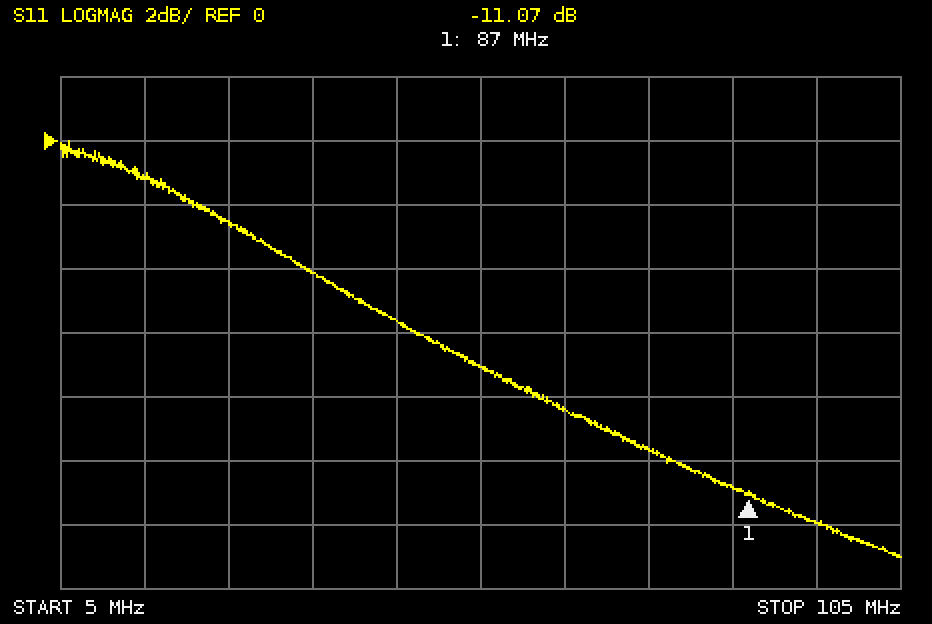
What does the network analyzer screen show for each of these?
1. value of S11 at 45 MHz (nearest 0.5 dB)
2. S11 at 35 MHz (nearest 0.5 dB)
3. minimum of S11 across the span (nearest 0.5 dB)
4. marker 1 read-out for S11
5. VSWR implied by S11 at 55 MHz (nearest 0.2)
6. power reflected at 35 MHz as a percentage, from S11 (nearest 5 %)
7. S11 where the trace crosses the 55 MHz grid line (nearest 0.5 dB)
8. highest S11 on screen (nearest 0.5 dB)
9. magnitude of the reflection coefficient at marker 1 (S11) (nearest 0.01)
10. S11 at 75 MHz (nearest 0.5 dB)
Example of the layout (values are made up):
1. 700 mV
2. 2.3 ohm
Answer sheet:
1. -5.5 dB
2. -4.0 dB
3. -13.0 dB
4. -11.07 dB
5. 2.6
6. 40 %
7. -7.0 dB
8. 0.0 dB
9. 0.28
10. -9.5 dB
